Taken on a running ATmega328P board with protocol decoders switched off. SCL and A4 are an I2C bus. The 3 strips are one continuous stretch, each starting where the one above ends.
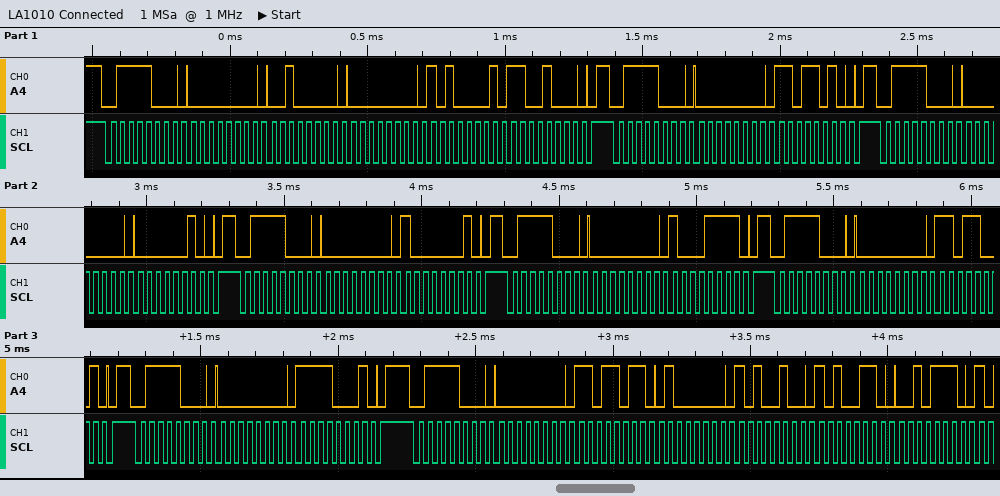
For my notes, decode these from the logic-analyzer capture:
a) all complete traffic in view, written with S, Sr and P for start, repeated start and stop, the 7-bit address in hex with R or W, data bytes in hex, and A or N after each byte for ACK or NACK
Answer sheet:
S 3CW A 00 A 20 A 00 A A1 A C8 A P S 3CW A 00 A DA A P S 3CW A 00 A 02 A P S 3CW A 00 A 81 A P S 3CW A 00 A 8F A P S 3CW A 00 A D9 A P S 3CW A 00 A F1 A P S 3CW A 00 A DB A 40 A A4 A A6 A 2E A
